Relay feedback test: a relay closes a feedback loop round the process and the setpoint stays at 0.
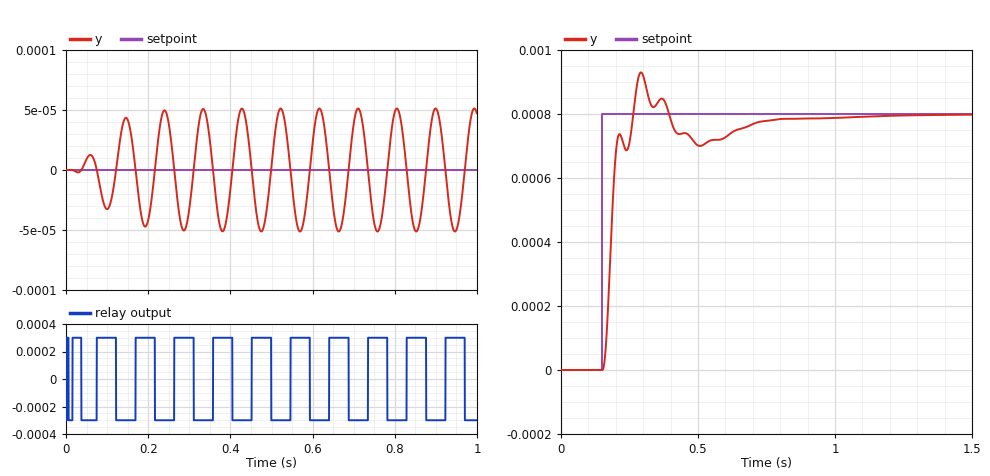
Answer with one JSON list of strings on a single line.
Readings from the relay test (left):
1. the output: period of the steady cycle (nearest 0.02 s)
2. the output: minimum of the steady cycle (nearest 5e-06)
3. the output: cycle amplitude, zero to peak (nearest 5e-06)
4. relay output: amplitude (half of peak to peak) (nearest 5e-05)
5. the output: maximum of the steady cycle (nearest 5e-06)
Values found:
["0.10 s", "-0.000050", "0.000050", "0.00030", "0.000050"]
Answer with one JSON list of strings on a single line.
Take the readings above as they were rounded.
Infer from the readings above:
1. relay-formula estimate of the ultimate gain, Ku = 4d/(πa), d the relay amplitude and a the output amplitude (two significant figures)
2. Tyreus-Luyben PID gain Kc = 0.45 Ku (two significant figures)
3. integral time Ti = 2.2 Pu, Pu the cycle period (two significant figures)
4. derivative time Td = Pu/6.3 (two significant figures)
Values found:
["7.6", "3.4", "0.22 s", "0.016 s"]
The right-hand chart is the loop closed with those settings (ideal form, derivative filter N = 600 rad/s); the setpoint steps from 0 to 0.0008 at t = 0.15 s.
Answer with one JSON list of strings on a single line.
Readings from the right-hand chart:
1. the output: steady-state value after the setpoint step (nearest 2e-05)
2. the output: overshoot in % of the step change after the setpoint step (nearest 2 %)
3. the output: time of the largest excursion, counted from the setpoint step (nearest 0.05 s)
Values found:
["0.00080", "16 %", "0.15 s"]
